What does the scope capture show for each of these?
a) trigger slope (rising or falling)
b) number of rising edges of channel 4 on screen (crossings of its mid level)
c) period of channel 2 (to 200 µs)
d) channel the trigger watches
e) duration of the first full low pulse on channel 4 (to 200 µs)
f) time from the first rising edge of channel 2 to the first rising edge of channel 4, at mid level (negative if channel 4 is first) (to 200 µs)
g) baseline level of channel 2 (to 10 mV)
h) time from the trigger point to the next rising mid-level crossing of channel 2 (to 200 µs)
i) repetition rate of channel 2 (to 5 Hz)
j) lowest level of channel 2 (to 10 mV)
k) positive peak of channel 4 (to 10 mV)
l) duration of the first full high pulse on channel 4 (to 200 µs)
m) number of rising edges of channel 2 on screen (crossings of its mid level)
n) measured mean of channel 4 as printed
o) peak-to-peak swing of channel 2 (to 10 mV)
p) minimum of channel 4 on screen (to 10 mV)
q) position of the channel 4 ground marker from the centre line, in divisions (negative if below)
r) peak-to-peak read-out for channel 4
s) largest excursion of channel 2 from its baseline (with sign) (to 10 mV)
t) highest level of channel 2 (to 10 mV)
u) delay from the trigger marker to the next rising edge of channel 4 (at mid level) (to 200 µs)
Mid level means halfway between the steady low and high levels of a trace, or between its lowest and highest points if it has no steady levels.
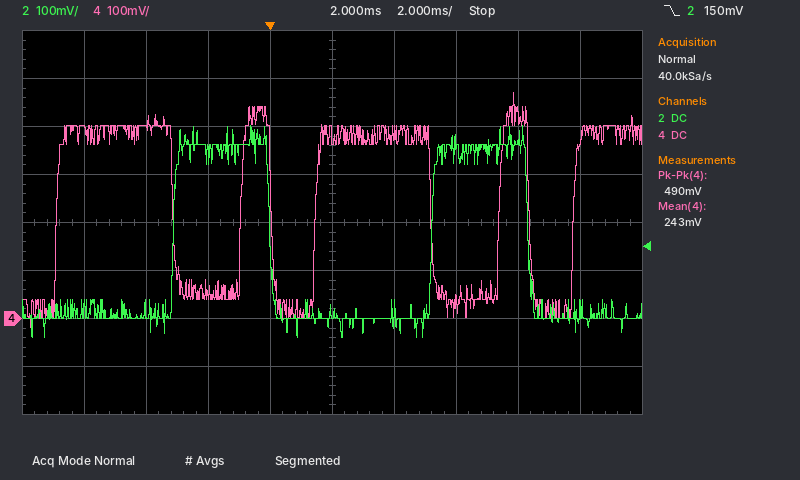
falling
5
8.4 ms
channel 2
2.2 ms
-3.8 ms
0 mV
5.2 ms
120 Hz
-40 mV
470 mV
3.8 ms
2
243 mV
440 mV
-20 mV
-2.0 div
490 mV
+400 mV
400 mV
1.4 ms
